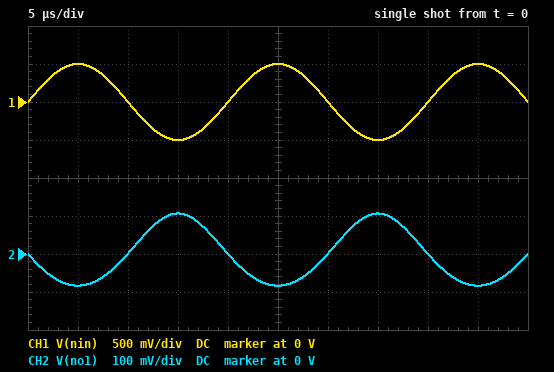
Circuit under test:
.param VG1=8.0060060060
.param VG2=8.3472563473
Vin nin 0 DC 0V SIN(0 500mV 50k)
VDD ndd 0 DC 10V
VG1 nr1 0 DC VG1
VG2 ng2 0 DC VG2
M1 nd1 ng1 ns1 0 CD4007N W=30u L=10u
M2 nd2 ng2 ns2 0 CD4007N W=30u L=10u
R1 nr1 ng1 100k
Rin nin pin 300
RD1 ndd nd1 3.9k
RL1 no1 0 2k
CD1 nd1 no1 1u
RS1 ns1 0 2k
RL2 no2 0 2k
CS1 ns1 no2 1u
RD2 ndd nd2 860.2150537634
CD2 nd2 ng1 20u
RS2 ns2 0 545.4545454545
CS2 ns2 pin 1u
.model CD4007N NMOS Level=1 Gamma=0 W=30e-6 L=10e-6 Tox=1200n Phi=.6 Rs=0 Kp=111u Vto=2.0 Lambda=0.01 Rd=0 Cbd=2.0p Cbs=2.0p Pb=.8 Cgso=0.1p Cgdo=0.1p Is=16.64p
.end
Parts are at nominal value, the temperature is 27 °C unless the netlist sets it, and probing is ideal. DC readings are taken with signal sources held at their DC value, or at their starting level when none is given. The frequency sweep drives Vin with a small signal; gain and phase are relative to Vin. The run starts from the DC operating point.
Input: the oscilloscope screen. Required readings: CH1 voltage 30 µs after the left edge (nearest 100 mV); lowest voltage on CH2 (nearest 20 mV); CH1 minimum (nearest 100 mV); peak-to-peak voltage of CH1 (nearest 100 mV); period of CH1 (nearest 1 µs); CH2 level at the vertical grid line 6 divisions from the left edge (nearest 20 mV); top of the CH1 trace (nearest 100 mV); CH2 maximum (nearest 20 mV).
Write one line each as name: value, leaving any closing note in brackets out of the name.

CH1 voltage 30 µs after the left edge: 0 V
lowest voltage on CH2: -80 mV
CH1 minimum: -500 mV
peak-to-peak voltage of CH1: 1.0 V
period of CH1: 20 µs
CH2 level at the vertical grid line 6 divisions from the left edge: 0 V
top of the CH1 trace: 500 mV
CH2 maximum: 100 mV
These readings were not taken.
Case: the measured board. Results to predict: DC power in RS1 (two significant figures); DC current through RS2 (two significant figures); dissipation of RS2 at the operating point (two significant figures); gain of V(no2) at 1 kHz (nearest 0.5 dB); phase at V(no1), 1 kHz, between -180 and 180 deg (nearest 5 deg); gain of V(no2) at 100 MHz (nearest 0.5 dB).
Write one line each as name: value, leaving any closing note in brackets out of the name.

DC power in RS1: 3.9 mW
DC current through RS2: 3.5 mA
dissipation of RS2 at the operating point: 6.6 mW
gain of V(no2) at 1 kHz: -17.5 dB
phase at V(no1), 1 kHz, between -180 and 180 deg: -160 deg
gain of V(no2) at 100 MHz: -17.5 dB
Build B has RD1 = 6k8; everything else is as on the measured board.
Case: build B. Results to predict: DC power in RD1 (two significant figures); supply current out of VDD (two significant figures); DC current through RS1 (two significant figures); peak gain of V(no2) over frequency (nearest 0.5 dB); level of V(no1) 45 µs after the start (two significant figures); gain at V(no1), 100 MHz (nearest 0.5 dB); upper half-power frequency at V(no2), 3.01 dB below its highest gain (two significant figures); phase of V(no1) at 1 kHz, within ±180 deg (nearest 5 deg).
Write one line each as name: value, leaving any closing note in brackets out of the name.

DC power in RD1: 7.3 mW
supply current out of VDD: 4.5 mA
DC current through RS1: 1.0 mA
peak gain of V(no2) over frequency: -26.0 dB
level of V(no1) 45 µs after the start: -35 mV
gain at V(no1), 100 MHz: -23.5 dB
upper half-power frequency at V(no2), 3.01 dB below its highest gain: 280 MHz
phase of V(no1) at 1 kHz, within ±180 deg: -160 deg
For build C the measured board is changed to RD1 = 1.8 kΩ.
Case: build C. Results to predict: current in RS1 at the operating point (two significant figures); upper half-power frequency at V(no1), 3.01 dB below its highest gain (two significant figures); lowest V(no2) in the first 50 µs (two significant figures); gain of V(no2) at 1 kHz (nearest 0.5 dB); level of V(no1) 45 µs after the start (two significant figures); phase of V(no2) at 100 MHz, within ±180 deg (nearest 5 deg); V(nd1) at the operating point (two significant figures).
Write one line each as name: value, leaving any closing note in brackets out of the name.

current in RS1 at the operating point: 1.5 mA
upper half-power frequency at V(no1), 3.01 dB below its highest gain: 280 MHz
lowest V(no2) in the first 50 µs: -170 mV
gain of V(no2) at 1 kHz: -10.0 dB
level of V(no1) 45 µs after the start: -150 mV
phase of V(no2) at 100 MHz, within ±180 deg: -40 deg
V(nd1) at the operating point: 7.3 V
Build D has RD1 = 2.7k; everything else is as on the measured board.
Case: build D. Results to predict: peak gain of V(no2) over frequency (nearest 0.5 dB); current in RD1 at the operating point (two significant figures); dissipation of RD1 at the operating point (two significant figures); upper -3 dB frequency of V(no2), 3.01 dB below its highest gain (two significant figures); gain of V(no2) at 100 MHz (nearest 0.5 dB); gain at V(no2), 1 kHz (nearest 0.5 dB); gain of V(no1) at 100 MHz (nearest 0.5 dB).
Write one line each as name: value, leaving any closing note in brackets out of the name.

peak gain of V(no2) over frequency: -10.0 dB
current in RD1 at the operating point: 1.5 mA
dissipation of RD1 at the operating point: 6.2 mW
upper -3 dB frequency of V(no2), 3.01 dB below its highest gain: 200 MHz
gain of V(no2) at 100 MHz: -11.0 dB
gain at V(no2), 1 kHz: -10.5 dB
gain of V(no1) at 100 MHz: -9.5 dB
